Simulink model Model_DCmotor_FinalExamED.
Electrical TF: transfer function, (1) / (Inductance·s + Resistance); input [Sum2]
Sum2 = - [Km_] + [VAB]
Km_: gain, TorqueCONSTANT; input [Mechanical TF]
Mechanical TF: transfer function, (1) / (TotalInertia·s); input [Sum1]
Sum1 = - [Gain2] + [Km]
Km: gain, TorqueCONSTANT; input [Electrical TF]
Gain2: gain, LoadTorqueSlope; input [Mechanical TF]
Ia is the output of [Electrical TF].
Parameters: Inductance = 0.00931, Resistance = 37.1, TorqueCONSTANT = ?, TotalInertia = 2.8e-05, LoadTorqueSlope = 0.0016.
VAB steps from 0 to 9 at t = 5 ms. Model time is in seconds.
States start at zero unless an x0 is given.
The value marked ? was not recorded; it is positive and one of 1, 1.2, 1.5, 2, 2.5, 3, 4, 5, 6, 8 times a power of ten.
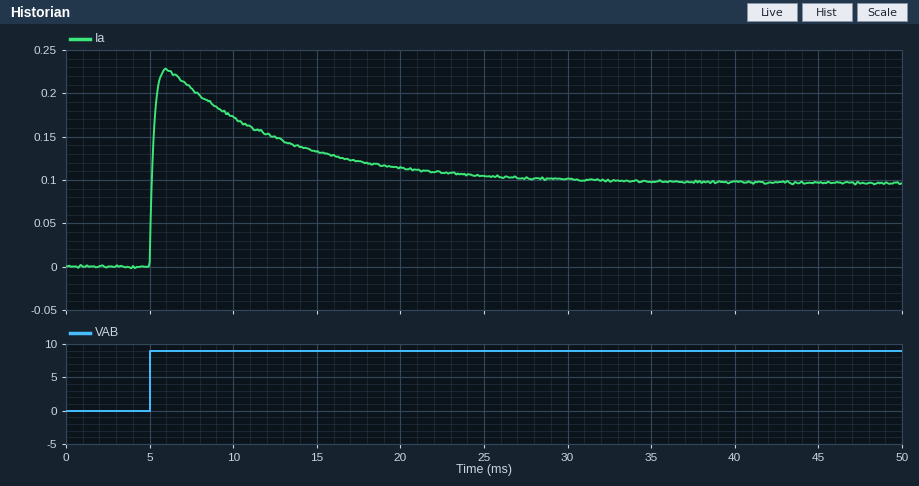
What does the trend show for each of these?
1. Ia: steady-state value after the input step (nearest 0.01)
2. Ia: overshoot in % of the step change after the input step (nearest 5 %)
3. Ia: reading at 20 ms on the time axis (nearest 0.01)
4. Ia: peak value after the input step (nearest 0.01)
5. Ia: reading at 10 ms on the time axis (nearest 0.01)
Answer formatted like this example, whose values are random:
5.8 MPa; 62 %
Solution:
0.10; 135 %; 0.11; 0.23; 0.17
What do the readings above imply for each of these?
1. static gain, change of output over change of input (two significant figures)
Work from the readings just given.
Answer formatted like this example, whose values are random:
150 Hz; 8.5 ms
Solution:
0.011
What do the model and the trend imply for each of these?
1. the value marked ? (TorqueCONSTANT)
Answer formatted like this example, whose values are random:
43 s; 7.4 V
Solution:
0.3
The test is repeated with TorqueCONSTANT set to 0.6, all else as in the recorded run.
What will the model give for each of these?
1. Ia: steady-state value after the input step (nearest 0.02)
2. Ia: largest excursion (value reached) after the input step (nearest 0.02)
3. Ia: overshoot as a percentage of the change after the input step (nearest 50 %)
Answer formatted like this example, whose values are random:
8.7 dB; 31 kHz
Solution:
0.04; 0.20; 500 %
